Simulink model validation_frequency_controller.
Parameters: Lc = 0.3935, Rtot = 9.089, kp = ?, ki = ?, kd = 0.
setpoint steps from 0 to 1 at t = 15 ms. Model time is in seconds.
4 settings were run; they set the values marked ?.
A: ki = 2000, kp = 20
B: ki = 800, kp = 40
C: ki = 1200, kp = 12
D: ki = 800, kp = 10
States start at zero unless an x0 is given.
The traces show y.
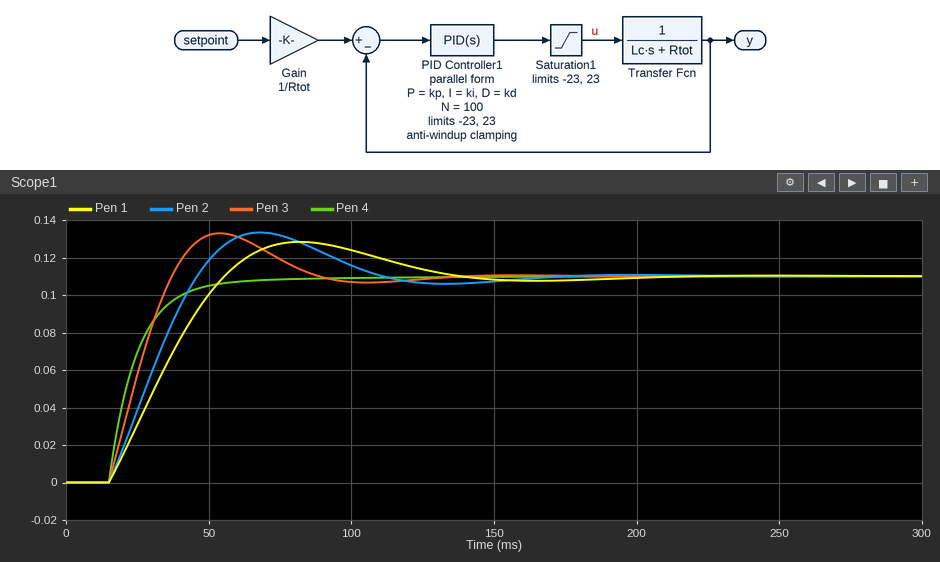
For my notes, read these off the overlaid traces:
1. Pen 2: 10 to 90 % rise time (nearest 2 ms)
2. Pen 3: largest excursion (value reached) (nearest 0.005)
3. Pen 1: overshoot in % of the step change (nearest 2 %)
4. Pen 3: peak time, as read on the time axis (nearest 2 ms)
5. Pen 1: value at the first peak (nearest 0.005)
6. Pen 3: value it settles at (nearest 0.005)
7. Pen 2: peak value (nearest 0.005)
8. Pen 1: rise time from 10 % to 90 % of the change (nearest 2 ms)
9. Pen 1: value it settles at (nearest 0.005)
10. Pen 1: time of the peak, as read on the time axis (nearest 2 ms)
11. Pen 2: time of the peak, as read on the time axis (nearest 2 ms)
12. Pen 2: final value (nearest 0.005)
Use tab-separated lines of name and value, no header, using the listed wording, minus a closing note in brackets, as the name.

Pen 2: 10 to 90 % rise time	24 ms
Pen 3: largest excursion (value reached)	0.135
Pen 1: overshoot in % of the step change	16 %
Pen 3: peak time, as read on the time axis	54 ms
Pen 1: value at the first peak	0.130
Pen 3: value it settles at	0.110
Pen 2: peak value	0.135
Pen 1: rise time from 10 % to 90 % of the change	30 ms
Pen 1: value it settles at	0.110
Pen 1: time of the peak, as read on the time axis	82 ms
Pen 2: time of the peak, as read on the time axis	68 ms
Pen 2: final value	0.110
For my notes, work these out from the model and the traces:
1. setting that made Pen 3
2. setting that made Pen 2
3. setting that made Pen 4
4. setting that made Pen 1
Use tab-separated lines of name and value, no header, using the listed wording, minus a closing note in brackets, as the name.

setting that made Pen 3	A
setting that made Pen 2	C
setting that made Pen 4	B
setting that made Pen 1	D
